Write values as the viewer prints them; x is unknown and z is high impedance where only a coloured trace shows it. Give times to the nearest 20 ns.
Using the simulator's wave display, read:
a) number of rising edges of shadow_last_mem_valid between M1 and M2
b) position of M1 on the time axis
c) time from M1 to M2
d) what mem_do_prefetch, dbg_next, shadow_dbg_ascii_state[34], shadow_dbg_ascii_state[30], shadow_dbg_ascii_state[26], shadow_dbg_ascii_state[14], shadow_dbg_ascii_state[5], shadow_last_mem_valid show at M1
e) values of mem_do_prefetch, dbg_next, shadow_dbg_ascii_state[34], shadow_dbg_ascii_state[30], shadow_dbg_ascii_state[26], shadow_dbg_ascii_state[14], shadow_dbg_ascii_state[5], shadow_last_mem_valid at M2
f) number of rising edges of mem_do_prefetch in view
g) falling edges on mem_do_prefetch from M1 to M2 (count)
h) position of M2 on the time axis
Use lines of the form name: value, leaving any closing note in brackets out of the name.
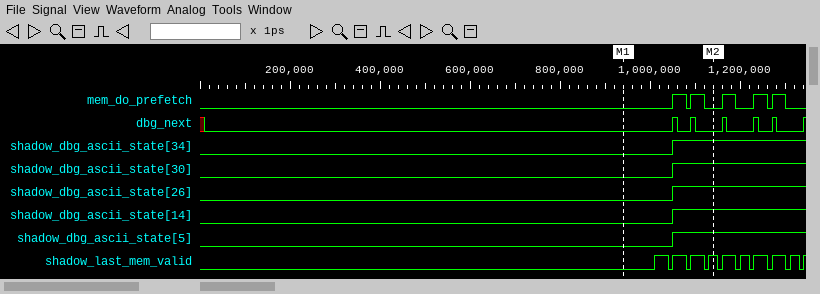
number of rising edges of shadow_last_mem_valid between M1 and M2: 4
position of M1 on the time axis: 940 ns
time from M1 to M2: 200 ns
what mem_do_prefetch, dbg_next, shadow_dbg_ascii_state[34], shadow_dbg_ascii_state[30], shadow_dbg_ascii_state[26], shadow_dbg_ascii_state[14], shadow_dbg_ascii_state[5], shadow_last_mem_valid show at M1: mem_do_prefetch=0, dbg_next=0, shadow_dbg_ascii_state[34]=0, shadow_dbg_ascii_state[30]=0, shadow_dbg_ascii_state[26]=0, shadow_dbg_ascii_state[14]=0, shadow_dbg_ascii_state[5]=0, shadow_last_mem_valid=0
values of mem_do_prefetch, dbg_next, shadow_dbg_ascii_state[34], shadow_dbg_ascii_state[30], shadow_dbg_ascii_state[26], shadow_dbg_ascii_state[14], shadow_dbg_ascii_state[5], shadow_last_mem_valid at M2: mem_do_prefetch=0, dbg_next=0, shadow_dbg_ascii_state[34]=1, shadow_dbg_ascii_state[30]=1, shadow_dbg_ascii_state[26]=1, shadow_dbg_ascii_state[14]=1, shadow_dbg_ascii_state[5]=1, shadow_last_mem_valid=1
number of rising edges of mem_do_prefetch in view: 5
falling edges on mem_do_prefetch from M1 to M2: 2
position of M2 on the time axis: 1140 ns
